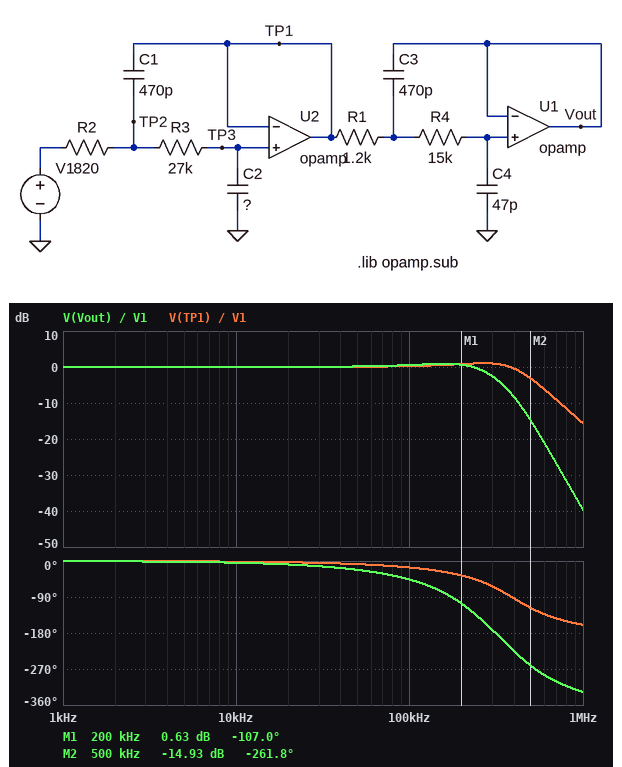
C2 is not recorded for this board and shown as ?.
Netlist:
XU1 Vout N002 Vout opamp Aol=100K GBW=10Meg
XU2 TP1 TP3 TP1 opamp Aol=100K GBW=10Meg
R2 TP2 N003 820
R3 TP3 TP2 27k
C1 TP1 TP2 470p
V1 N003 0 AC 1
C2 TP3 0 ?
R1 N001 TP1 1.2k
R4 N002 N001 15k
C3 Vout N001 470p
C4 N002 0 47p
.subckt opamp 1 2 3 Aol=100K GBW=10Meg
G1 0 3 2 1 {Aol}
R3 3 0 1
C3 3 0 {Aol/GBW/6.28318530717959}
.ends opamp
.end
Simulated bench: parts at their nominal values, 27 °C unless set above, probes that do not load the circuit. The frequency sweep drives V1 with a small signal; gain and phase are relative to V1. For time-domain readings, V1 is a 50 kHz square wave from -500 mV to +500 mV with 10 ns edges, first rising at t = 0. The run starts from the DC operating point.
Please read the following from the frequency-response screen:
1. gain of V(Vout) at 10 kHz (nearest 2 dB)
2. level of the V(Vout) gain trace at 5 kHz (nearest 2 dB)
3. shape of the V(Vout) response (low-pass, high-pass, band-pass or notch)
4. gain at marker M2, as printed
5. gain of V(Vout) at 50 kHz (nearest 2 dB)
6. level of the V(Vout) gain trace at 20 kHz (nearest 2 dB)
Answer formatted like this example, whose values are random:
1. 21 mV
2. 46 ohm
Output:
1. 0 dB
2. 0 dB
3. low-pass
4. -14.93 dB
5. 0 dB
6. 0 dB
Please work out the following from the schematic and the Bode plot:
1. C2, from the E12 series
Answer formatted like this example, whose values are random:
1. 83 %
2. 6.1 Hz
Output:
1. 15 pF
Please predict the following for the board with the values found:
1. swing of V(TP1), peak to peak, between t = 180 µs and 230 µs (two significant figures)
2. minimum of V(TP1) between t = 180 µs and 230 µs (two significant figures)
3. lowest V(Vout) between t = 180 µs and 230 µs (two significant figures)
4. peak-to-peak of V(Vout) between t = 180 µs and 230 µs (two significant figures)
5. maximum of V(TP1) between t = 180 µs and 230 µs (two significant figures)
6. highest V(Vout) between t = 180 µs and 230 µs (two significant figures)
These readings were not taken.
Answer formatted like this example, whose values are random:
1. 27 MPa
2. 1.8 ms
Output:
1. 1.3 V
2. -650 mV
3. -660 mV
4. 1.3 V
5. 650 mV
6. 660 mV
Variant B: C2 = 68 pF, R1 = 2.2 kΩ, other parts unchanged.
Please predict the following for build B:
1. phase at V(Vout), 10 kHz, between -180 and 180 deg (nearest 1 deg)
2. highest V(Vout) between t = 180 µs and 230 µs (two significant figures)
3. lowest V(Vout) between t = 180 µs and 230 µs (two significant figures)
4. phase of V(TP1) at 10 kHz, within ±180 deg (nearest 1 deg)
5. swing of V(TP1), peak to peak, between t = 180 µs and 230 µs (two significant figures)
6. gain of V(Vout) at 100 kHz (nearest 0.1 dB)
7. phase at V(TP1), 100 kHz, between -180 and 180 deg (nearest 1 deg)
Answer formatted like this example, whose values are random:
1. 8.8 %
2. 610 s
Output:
1. -10 deg
2. 510 mV
3. -510 mV
4. -7 deg
5. 1.0 V
6. -1.6 dB
7. -59 deg
